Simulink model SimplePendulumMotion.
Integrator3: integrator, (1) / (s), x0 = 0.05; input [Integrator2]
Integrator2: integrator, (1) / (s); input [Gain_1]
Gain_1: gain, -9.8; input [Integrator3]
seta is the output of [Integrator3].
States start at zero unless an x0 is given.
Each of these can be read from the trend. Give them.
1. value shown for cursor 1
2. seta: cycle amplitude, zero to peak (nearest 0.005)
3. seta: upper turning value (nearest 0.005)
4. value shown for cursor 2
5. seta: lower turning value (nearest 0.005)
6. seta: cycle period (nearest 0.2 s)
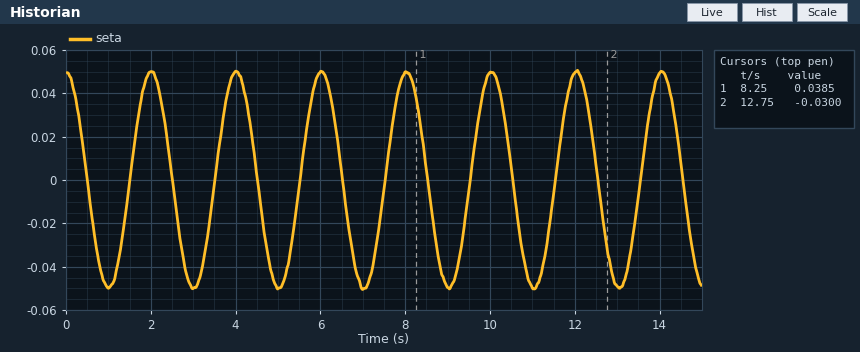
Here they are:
0.0385
0.050
0.050
-0.0300
-0.050
2.0 s
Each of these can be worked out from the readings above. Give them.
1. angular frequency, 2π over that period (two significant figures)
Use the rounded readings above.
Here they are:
3.1 rad/s
